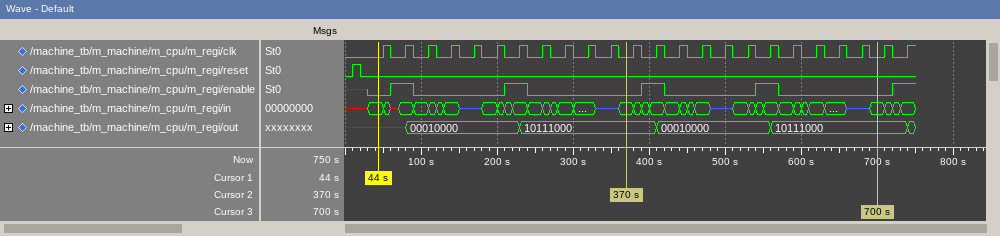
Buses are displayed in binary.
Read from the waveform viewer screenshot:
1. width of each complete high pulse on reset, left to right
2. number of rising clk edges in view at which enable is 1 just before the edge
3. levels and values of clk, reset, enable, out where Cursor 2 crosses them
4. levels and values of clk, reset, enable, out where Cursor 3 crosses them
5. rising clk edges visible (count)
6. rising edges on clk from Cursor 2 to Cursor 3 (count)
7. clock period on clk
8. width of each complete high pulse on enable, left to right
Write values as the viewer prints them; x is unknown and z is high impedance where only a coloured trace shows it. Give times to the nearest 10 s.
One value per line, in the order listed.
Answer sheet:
10 s
5
clk=0, reset=0, enable=0, out=10111000
clk=0, reset=0, enable=0, out=10111000
24
11
30 s
30 s, 30 s, 30 s, 30 s
